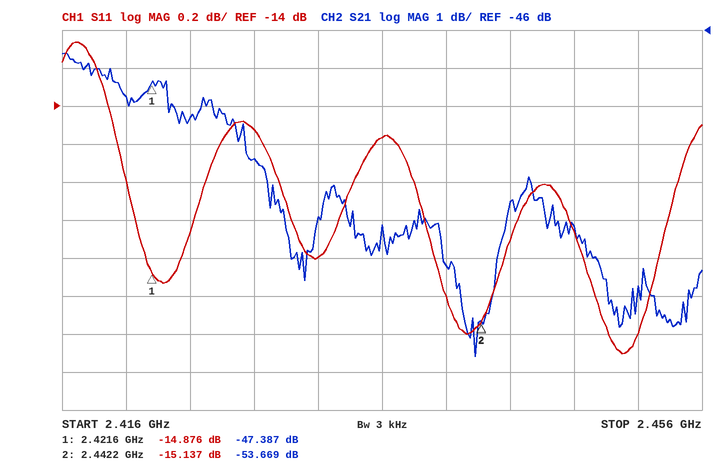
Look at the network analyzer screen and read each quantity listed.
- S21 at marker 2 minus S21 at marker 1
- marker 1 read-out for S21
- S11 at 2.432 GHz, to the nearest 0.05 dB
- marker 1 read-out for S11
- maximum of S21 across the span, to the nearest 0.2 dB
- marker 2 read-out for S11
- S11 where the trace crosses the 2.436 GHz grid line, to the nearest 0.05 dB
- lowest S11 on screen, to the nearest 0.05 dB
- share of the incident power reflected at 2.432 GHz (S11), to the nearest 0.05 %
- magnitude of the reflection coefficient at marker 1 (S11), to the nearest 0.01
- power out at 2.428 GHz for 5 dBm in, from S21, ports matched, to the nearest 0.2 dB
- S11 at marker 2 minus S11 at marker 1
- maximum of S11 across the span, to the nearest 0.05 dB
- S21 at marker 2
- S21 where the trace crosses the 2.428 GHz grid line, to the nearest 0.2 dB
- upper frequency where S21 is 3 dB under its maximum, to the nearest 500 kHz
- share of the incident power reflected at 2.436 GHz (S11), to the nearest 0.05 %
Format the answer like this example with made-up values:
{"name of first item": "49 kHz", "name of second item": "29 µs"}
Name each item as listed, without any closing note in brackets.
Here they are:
{"S21 at marker 2 minus S21 at marker 1": "-6.282 dB", "marker 1 read-out for S21": "-47.387 dB", "S11 at 2.432 GHz, to the nearest 0.05 dB": "-14.80 dB", "marker 1 read-out for S11": "-14.876 dB", "maximum of S21 across the span, to the nearest 0.2 dB": "-46.6 dB", "marker 2 read-out for S11": "-15.137 dB", "S11 where the trace crosses the 2.436 GHz grid line, to the nearest 0.05 dB": "-14.15 dB", "lowest S11 on screen, to the nearest 0.05 dB": "-15.30 dB", "share of the incident power reflected at 2.432 GHz (S11), to the nearest 0.05 %": "3.30 %", "magnitude of the reflection coefficient at marker 1 (S11), to the nearest 0.01": "0.18", "power out at 2.428 GHz for 5 dBm in, from S21, ports matched, to the nearest 0.2 dB": "-44.4 dBm", "S11 at marker 2 minus S11 at marker 1": "-0.261 dB", "maximum of S11 across the span, to the nearest 0.05 dB": "-13.65 dB", "S21 at marker 2": "-53.669 dB", "S21 where the trace crosses the 2.428 GHz grid line, to the nearest 0.2 dB": "-49.4 dB", "upper frequency where S21 is 3 dB under its maximum, to the nearest 500 kHz": "2.4285 GHz", "share of the incident power reflected at 2.436 GHz (S11), to the nearest 0.05 %": "3.85 %"}
